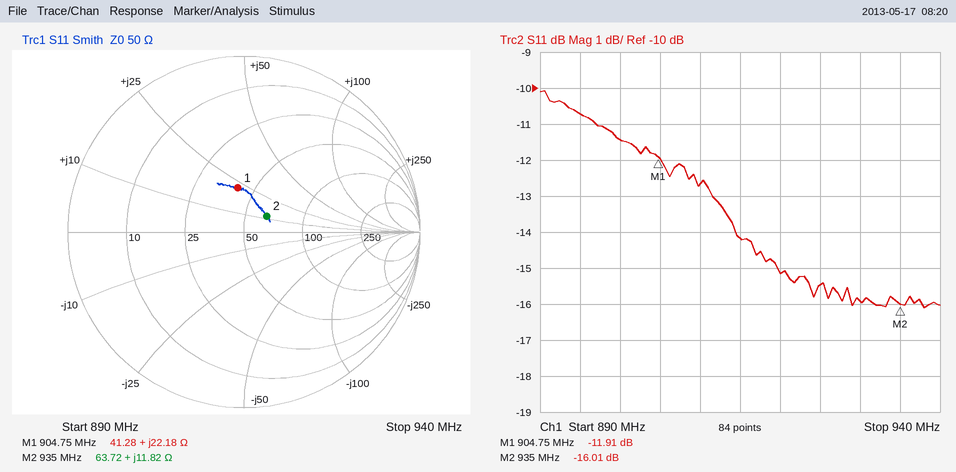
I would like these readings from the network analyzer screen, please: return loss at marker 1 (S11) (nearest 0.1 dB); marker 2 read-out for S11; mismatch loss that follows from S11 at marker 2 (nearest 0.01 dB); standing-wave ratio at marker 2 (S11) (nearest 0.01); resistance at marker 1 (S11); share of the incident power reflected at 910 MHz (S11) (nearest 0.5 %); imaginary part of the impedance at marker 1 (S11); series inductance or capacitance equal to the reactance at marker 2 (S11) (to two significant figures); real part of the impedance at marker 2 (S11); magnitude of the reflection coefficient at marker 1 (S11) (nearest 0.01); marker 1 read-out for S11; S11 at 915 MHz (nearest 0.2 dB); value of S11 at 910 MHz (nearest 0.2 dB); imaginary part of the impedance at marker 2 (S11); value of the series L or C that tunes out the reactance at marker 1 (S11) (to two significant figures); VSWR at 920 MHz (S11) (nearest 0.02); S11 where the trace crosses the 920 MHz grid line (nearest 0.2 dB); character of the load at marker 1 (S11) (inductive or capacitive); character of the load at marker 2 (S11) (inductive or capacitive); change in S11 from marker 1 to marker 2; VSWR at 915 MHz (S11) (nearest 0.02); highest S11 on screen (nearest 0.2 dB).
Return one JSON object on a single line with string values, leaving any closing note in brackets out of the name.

{"return loss at marker 1 (S11)": "11.9 dB", "marker 2 read-out for S11": "-16.01 dB", "mismatch loss that follows from S11 at marker 2": "0.11 dB", "standing-wave ratio at marker 2 (S11)": "1.38", "resistance at marker 1": "41.28 Ω", "share of the incident power reflected at 910 MHz (S11)": "5.5 %", "imaginary part of the impedance at marker 1": "+22.18 Ω", "series inductance or capacitance equal to the reactance at marker 2 (S11)": "2.0 nH", "real part of the impedance at marker 2": "63.72 Ω", "magnitude of the reflection coefficient at marker 1 (S11)": "0.25", "marker 1 read-out for S11": "-11.91 dB", "S11 at 915 MHz": "-14.2 dB", "value of S11 at 910 MHz": "-12.6 dB", "imaginary part of the impedance at marker 2": "+11.82 Ω", "value of the series L or C that tunes out the reactance at marker 1 (S11)": "7.9 pF", "VSWR at 920 MHz (S11)": "1.42", "S11 where the trace crosses the 920 MHz grid line": "-15.2 dB", "character of the load at marker 1 (S11)": "inductive", "character of the load at marker 2 (S11)": "inductive", "change in S11 from marker 1 to marker 2": "-4.10 dB", "VSWR at 915 MHz (S11)": "1.48", "highest S11 on screen": "-10.0 dB"}
